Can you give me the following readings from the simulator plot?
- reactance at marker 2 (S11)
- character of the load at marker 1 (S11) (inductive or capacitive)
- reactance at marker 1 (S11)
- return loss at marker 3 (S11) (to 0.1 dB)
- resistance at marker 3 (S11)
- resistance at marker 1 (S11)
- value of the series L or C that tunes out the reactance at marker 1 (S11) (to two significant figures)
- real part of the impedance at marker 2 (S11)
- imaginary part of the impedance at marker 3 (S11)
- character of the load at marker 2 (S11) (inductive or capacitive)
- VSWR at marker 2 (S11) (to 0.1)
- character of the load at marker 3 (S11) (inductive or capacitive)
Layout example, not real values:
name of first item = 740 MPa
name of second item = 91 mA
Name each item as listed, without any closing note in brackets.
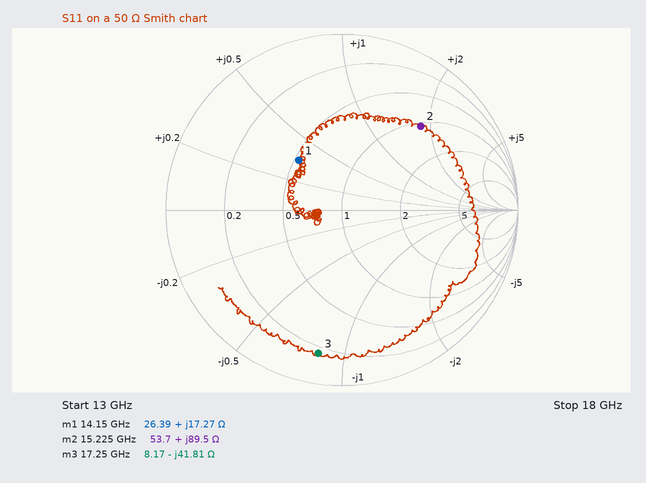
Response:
reactance at marker 2 = +89.5 Ω
character of the load at marker 1 (S11) = inductive
reactance at marker 1 = +17.27 Ω
return loss at marker 3 (S11) = 1.7 dB
resistance at marker 3 = 8.17 Ω
resistance at marker 1 = 26.39 Ω
value of the series L or C that tunes out the reactance at marker 1 (S11) = 650 fF
real part of the impedance at marker 2 = 53.7 Ω
imaginary part of the impedance at marker 3 = -41.81 Ω
character of the load at marker 2 (S11) = inductive
VSWR at marker 2 (S11) = 4.8
character of the load at marker 3 (S11) = capacitive
